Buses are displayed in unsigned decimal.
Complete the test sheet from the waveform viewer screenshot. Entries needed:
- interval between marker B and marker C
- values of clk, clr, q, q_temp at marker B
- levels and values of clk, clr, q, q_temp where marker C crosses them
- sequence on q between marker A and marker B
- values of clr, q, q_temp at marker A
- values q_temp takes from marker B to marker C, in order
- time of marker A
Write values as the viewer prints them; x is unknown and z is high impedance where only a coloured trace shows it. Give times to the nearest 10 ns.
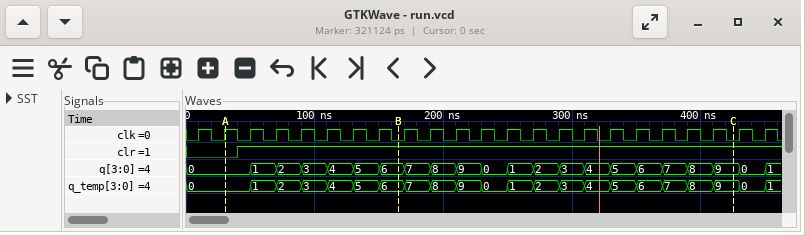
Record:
260 ns
clk=0, clr=1, q=6, q_temp=6
clk=0, clr=1, q=9, q_temp=9
0, 1, 2, 3, 4, 5, 6
clr=0, q=0, q_temp=0
6, 7, 8, 9, 0, 1, 2, 3, 4, 5, 6, 7, 8, 9
30 ns
